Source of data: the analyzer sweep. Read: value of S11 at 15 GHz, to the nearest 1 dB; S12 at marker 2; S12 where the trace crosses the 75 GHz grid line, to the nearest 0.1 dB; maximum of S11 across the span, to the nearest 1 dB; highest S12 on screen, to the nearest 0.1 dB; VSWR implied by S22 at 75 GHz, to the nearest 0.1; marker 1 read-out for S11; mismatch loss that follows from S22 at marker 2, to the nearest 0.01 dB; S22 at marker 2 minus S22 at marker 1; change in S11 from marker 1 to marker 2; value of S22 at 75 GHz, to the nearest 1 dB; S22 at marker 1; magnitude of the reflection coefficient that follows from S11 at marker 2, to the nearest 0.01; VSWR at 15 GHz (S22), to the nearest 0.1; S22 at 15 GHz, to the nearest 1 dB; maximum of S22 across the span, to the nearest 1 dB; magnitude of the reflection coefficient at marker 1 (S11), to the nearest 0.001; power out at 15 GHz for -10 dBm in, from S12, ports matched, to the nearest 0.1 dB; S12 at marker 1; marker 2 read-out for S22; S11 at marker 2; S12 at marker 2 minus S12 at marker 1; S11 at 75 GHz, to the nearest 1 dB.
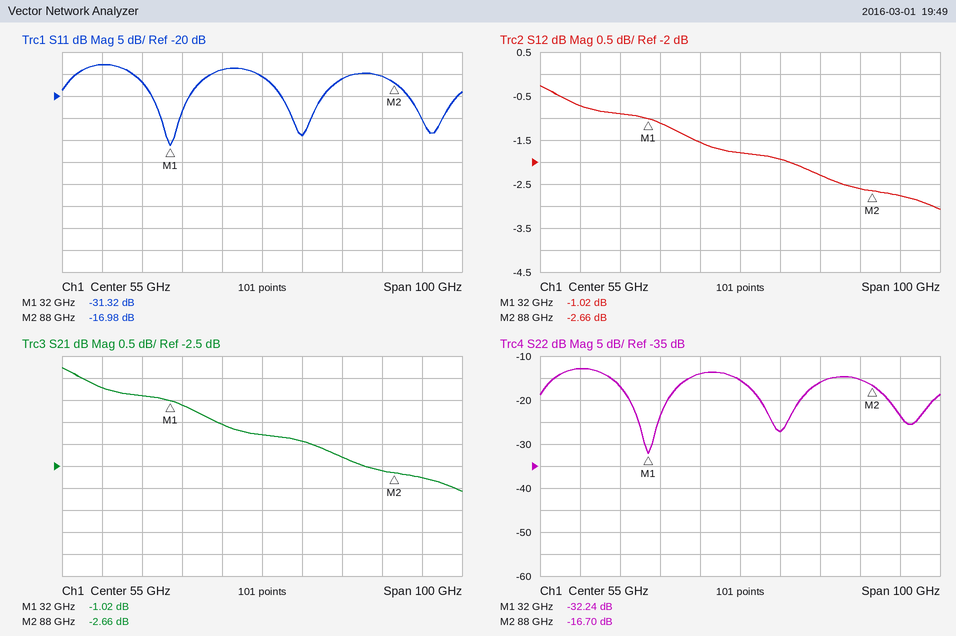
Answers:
-13 dB
-2.66 dB
-2.3 dB
-13 dB
-0.3 dB
1.4
-31.32 dB
0.09 dB
15.54 dB
14.34 dB
-16 dB
-32.24 dB
0.14
1.6
-13 dB
-13 dB
0.027
-10.7 dBm
-1.02 dB
-16.70 dB
-16.98 dB
-1.64 dB
-16 dB
